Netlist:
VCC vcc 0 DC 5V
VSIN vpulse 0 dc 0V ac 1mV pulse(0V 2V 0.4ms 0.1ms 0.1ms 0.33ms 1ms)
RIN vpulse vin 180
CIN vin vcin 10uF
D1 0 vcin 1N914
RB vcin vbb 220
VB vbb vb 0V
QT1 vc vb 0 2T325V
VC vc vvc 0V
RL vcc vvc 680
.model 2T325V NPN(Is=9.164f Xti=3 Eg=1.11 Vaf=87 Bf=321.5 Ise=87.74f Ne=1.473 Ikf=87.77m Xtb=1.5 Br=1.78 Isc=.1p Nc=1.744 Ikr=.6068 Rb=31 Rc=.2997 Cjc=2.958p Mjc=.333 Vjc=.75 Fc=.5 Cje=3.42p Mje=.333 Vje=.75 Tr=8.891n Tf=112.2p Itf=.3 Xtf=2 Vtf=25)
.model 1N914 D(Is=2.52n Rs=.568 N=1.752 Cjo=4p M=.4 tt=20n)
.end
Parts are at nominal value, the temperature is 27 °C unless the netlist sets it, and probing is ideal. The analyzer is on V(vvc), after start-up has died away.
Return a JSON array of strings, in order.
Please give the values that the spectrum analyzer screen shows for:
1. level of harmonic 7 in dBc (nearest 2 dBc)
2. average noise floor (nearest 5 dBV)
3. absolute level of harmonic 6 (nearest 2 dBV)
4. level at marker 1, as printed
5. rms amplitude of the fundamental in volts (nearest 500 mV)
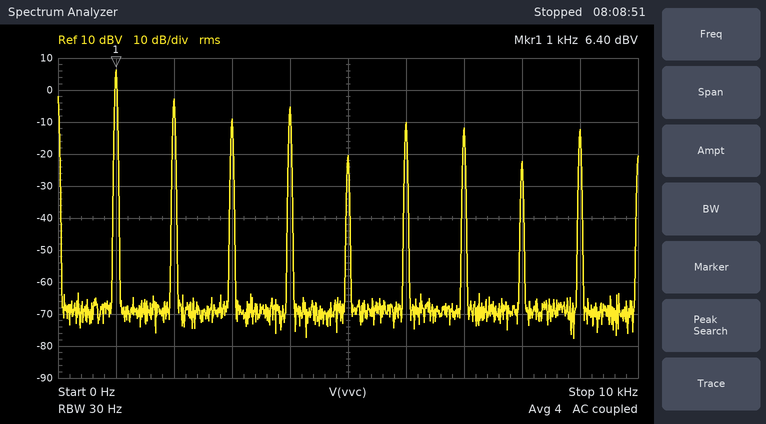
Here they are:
["-18 dBc", "-70 dBV", "-10 dBV", "6.40 dBV", "2.0 V"]
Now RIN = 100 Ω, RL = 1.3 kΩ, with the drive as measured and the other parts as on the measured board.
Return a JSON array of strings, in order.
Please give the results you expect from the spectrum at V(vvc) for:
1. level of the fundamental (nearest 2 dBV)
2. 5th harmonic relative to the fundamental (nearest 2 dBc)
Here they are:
["6 dBV", "-30 dBc"]
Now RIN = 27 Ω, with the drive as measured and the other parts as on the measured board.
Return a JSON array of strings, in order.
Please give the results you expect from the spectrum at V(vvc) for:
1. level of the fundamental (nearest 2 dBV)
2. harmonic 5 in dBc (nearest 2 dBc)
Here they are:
["6 dBV", "-36 dBc"]
